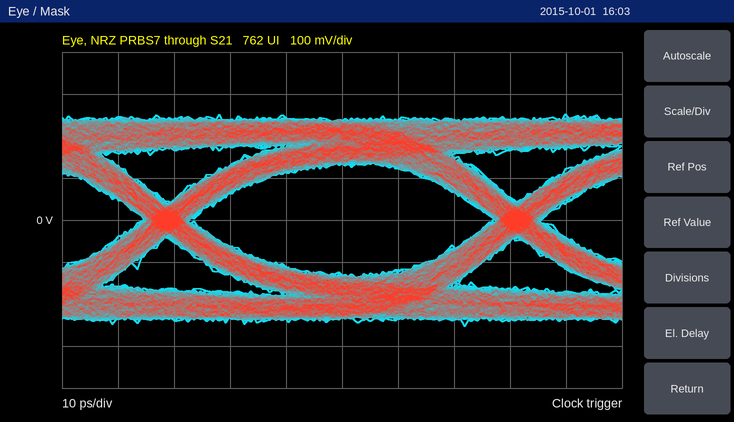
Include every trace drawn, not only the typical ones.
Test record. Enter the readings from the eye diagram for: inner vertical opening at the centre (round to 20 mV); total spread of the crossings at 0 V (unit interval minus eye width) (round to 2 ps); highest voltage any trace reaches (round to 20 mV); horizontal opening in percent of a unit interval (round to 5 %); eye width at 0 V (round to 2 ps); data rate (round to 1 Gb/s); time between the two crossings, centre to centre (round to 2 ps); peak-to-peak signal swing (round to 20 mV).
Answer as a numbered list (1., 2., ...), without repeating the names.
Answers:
1. 260 mV
2. 8 ps
3. 260 mV
4. 85 %
5. 54 ps
6. 16 Gb/s
7. 62 ps
8. 500 mV
